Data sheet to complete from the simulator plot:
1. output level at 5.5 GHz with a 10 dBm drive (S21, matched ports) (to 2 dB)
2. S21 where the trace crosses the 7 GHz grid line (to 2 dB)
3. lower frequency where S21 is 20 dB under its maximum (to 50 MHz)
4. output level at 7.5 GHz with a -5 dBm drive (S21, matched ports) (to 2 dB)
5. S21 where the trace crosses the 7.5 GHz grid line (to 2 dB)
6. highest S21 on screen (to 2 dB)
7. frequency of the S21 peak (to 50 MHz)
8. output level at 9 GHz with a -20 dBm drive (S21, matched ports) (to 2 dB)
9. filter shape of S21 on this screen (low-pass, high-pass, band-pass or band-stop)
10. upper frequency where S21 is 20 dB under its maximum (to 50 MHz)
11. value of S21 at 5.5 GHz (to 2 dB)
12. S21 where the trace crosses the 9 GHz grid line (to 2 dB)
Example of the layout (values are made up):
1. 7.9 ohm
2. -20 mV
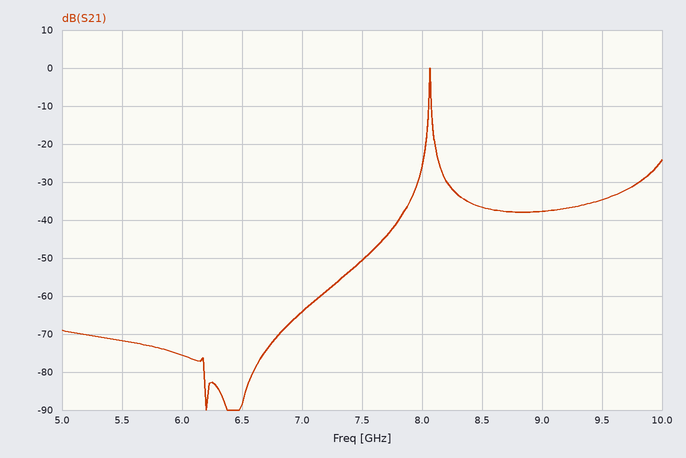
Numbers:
1. -62 dBm
2. -64 dB
3. 8.05 GHz
4. -56 dBm
5. -50 dB
6. 0 dB
7. 8.05 GHz
8. -58 dBm
9. band-pass
10. 8.10 GHz
11. -72 dB
12. -38 dB
